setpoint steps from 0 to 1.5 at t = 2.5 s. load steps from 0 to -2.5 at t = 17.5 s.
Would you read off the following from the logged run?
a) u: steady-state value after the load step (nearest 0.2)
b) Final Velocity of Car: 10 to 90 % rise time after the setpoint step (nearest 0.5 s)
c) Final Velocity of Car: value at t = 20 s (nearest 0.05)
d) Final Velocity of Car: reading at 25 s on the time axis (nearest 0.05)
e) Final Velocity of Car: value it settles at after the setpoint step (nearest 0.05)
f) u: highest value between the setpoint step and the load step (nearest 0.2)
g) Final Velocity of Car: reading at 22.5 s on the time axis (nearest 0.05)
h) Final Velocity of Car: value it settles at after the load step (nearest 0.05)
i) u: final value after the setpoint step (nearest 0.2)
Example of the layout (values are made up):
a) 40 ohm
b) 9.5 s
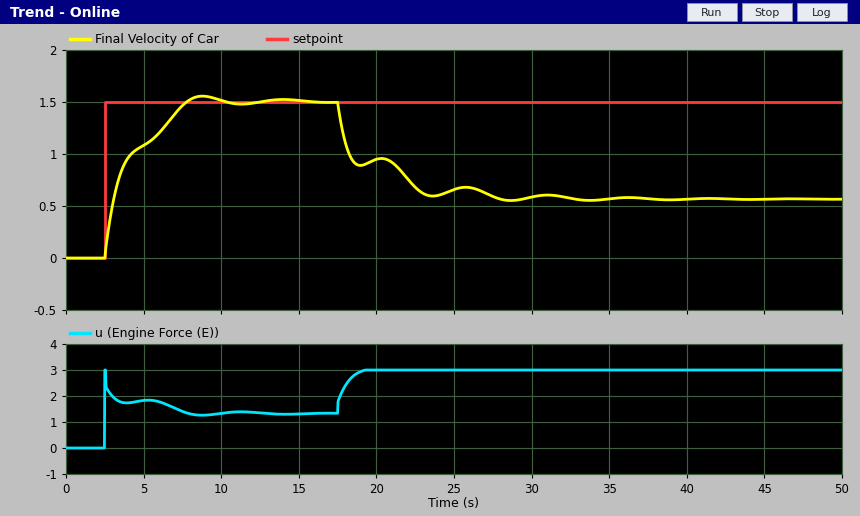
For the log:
a) 3.0
b) 4.0 s
c) 0.95
d) 0.65
e) 1.50
f) 3.0
g) 0.70
h) 0.55
i) 1.4
